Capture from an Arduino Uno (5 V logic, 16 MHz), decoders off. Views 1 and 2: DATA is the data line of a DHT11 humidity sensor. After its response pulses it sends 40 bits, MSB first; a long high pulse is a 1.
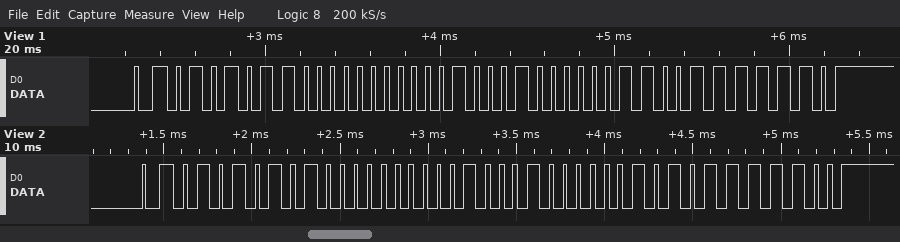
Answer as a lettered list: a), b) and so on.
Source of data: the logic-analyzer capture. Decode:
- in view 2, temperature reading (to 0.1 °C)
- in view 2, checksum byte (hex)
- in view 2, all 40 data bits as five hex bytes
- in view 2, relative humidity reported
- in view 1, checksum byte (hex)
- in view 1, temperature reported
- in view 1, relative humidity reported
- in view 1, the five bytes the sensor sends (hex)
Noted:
a) 34.5 °C
b) 0x7C
c) 55 00 22 05 7C
d) 85 %
e) 0x7E
f) 34.6 °C
g) 86 %
h) 56 00 22 06 7E
